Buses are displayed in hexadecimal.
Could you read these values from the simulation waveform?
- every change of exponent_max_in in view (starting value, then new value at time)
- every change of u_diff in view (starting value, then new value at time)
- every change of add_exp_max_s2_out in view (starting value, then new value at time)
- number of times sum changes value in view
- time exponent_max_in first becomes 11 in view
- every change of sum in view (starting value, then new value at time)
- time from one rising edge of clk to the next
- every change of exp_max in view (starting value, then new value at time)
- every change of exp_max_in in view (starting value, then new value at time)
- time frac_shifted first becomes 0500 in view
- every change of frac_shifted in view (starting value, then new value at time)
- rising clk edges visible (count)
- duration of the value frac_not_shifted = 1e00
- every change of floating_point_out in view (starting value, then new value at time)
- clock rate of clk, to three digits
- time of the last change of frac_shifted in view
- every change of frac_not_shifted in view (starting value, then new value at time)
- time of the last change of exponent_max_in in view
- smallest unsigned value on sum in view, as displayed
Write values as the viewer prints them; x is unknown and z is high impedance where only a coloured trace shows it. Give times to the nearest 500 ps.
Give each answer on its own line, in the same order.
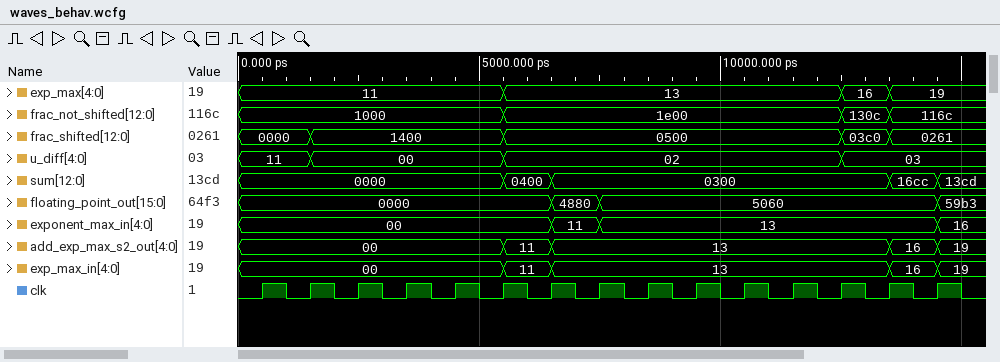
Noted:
00, 11 at 6500 ps, 13 at 7500 ps, 16 at 14500 ps
11, 00 at 1500 ps, 02 at 5500 ps, 03 at 12500 ps
00, 11 at 5500 ps, 13 at 6500 ps, 16 at 13500 ps, 19 at 14500 ps
4
6500 ps
0000, 0400 at 5500 ps, 0300 at 6500 ps, 16cc at 13500 ps, 13cd at 14500 ps
1000 ps
11, 13 at 5500 ps, 16 at 12500 ps, 19 at 13500 ps
00, 11 at 5500 ps, 13 at 6500 ps, 16 at 13500 ps, 19 at 14500 ps
5500 ps
0000, 1400 at 1500 ps, 0500 at 5500 ps, 03c0 at 12500 ps, 0261 at 13500 ps
15
7000 ps
0000, 4880 at 6500 ps, 5060 at 7500 ps, 59b3 at 14500 ps
1.00 GHz
13500 ps
1000, 1e00 at 5500 ps, 130c at 12500 ps, 116c at 13500 ps
14500 ps
0000
